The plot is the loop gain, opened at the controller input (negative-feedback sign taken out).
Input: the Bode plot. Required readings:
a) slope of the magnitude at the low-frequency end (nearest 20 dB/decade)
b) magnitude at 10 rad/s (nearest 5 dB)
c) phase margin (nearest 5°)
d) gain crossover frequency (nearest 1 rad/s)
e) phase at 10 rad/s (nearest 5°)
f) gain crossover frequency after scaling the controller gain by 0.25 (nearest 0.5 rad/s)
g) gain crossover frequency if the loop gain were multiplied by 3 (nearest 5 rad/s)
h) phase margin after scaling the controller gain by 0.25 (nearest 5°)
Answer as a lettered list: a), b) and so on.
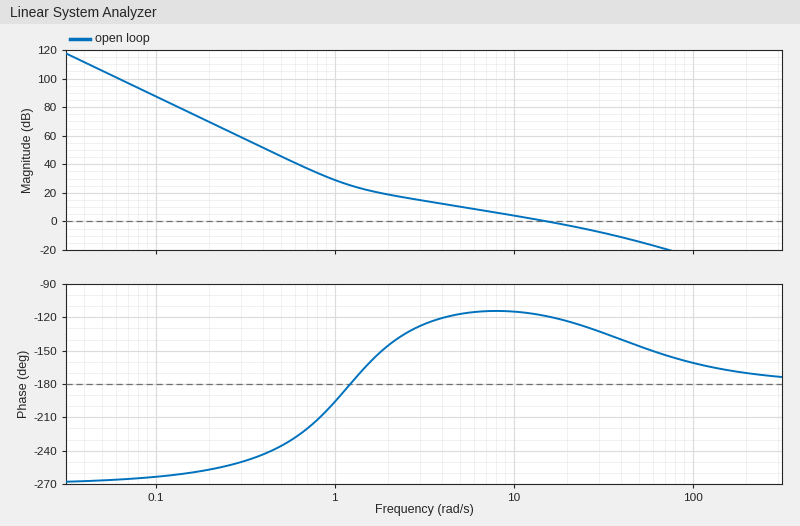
a) -60 dB/decade
b) 5 dB
c) 60°
d) 15 rad/s
e) -115°
f) 4.0 rad/s
g) 35 rad/s
h) 60°
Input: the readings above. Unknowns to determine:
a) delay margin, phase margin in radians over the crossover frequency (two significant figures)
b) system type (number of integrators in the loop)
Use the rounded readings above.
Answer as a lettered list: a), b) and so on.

a) 0.070 s
b) 3
